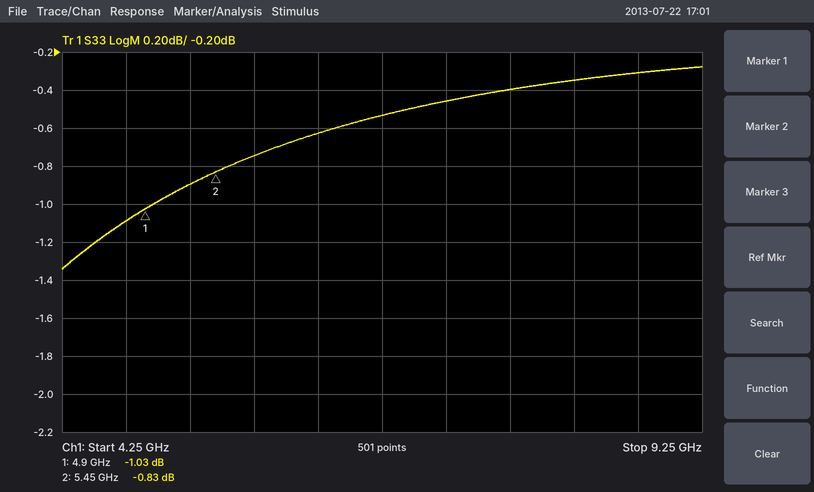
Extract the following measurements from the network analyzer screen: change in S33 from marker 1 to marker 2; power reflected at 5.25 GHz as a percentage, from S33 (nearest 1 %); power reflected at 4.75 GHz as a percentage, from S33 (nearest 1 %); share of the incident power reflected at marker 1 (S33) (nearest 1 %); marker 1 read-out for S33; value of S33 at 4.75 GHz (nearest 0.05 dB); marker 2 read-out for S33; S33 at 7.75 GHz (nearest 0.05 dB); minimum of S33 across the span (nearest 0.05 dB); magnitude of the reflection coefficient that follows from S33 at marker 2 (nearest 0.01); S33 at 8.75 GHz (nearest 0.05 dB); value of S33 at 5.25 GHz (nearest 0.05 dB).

0.20 dB
81 %
78 %
79 %
-1.03 dB
-1.10 dB
-0.83 dB
-0.40 dB
-1.35 dB
0.91
-0.30 dB
-0.90 dB
